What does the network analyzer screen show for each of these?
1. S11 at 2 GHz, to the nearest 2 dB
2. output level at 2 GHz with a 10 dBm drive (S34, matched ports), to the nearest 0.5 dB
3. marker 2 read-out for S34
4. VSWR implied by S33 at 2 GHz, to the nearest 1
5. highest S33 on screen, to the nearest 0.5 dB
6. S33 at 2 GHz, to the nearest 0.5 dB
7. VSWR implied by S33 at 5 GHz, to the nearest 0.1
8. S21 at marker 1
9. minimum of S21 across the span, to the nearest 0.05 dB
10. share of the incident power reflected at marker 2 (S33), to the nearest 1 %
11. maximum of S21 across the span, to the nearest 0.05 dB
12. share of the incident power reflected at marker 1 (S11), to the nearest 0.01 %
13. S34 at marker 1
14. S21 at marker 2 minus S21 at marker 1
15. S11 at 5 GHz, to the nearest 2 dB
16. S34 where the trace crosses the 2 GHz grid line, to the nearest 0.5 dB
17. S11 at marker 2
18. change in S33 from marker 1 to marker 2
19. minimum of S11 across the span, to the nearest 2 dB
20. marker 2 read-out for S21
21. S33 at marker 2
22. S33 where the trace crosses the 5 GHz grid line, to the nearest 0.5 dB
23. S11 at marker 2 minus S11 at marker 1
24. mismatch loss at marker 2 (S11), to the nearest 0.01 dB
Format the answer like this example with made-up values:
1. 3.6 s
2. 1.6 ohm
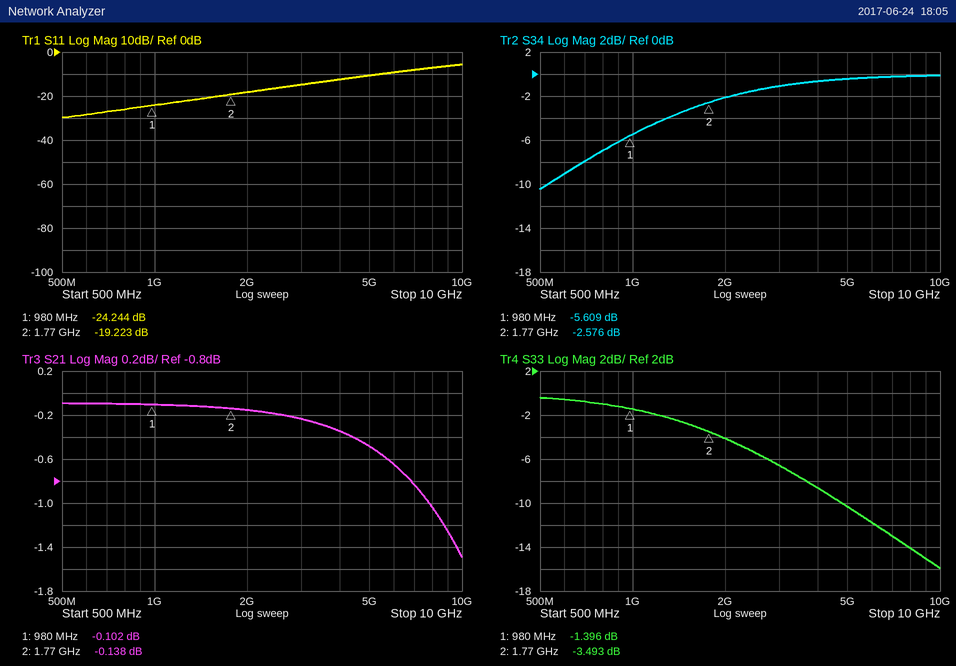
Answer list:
1. -18 dB
2. 8.0 dBm
3. -2.576 dB
4. 4
5. -0.5 dB
6. -4.0 dB
7. 1.9
8. -0.102 dB
9. -1.50 dB
10. 45 %
11. -0.10 dB
12. 0.38 %
13. -5.609 dB
14. -0.036 dB
15. -10 dB
16. -2.0 dB
17. -19.223 dB
18. -2.097 dB
19. -30 dB
20. -0.138 dB
21. -3.493 dB
22. -10.5 dB
23. 5.021 dB
24. 0.05 dB
